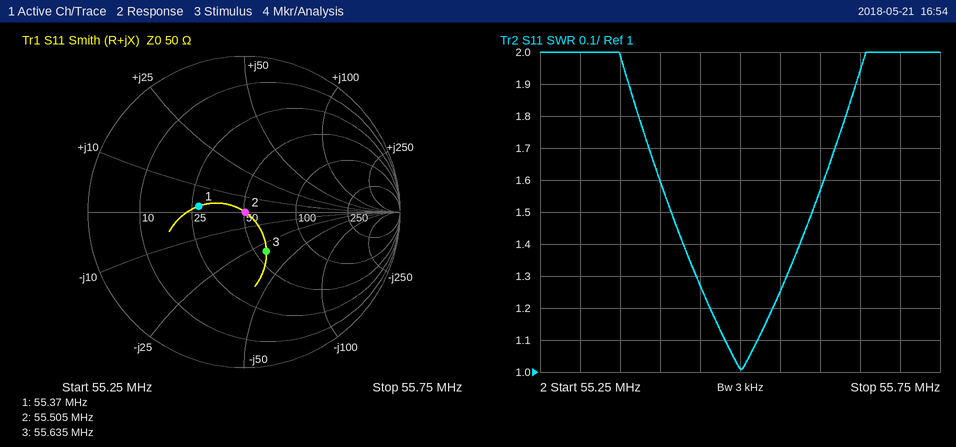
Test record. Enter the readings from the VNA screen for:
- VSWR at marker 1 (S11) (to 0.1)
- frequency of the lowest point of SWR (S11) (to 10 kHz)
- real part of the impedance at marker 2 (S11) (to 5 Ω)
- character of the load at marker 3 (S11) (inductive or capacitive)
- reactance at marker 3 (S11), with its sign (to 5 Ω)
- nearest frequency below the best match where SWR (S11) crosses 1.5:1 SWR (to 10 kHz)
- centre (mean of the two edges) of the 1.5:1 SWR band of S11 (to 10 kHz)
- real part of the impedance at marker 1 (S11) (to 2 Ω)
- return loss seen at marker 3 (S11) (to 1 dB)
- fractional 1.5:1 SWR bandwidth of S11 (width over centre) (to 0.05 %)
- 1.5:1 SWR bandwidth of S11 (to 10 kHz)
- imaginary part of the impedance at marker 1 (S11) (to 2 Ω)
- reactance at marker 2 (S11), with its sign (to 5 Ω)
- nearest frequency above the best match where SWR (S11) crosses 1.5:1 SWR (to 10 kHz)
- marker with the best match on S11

1.8
55.50 MHz
50 Ω
capacitive
-30 Ω
55.41 MHz
55.50 MHz
28 Ω
11 dB
0.30 %
180 kHz
+2 Ω
0 Ω
55.59 MHz
marker 2
